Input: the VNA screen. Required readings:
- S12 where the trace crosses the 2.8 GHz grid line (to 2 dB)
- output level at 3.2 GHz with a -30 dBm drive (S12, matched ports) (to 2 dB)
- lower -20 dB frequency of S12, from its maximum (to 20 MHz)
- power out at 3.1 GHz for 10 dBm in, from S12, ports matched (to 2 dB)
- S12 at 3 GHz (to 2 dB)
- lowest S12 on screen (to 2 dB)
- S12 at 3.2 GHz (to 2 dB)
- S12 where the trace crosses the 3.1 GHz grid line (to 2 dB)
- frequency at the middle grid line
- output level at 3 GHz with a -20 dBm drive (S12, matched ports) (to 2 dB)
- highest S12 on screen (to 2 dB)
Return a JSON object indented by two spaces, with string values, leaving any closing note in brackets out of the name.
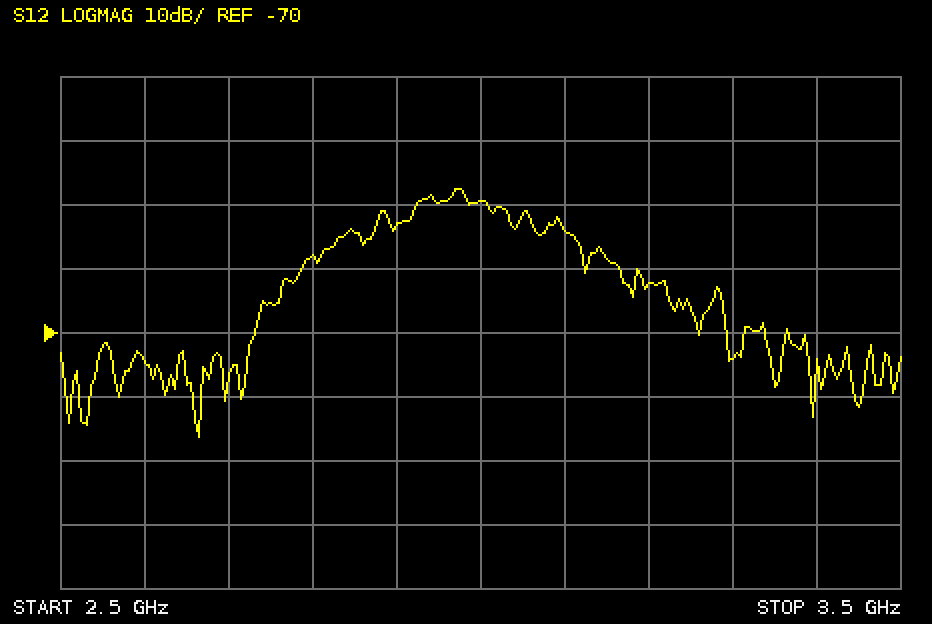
{
  "S12 where the trace crosses the 2.8 GHz grid line": "-58 dB",
  "output level at 3.2 GHz with a -30 dBm drive (S12, matched ports)": "-92 dBm",
  "lower -20 dB frequency of S12, from its maximum": "2.74 GHz",
  "power out at 3.1 GHz for 10 dBm in, from S12, ports matched": "-44 dBm",
  "S12 at 3 GHz": "-50 dB",
  "lowest S12 on screen": "-86 dB",
  "S12 at 3.2 GHz": "-62 dB",
  "S12 where the trace crosses the 3.1 GHz grid line": "-54 dB",
  "frequency at the middle grid line": "3 GHz",
  "output level at 3 GHz with a -20 dBm drive (S12, matched ports)": "-70 dBm",
  "highest S12 on screen": "-48 dB"
}
